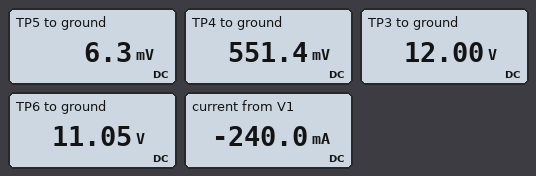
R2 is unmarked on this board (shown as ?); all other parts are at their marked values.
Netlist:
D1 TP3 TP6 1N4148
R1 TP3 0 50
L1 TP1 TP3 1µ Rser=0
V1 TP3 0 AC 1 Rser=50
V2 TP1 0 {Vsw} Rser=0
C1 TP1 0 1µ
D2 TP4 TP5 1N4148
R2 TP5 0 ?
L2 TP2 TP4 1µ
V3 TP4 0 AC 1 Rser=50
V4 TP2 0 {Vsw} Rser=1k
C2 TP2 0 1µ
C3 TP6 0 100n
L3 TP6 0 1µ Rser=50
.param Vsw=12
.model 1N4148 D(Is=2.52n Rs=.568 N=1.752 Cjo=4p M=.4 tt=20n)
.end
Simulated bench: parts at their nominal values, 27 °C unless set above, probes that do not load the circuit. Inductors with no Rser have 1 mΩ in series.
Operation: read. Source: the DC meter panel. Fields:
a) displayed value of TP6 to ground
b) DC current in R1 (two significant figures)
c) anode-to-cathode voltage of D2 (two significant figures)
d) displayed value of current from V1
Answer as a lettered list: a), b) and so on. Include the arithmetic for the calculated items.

a) 11.05 V
b) (12 V) / 50 Ω = 240 mA
c) 551.4 mV - 6.3 mV = 550 mV
d) -240.0 mA
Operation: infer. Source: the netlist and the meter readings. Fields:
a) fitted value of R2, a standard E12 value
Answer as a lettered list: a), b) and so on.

a) 15 Ω
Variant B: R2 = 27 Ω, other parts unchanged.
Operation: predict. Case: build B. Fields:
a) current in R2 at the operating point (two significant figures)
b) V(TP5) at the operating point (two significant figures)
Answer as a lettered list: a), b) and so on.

a) 390 µA
b) 11 mV
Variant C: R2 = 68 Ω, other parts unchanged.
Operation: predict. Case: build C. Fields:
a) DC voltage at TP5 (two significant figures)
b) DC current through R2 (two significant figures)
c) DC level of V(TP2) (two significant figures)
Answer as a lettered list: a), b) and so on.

a) 22 mV
b) 330 µA
c) 560 mV
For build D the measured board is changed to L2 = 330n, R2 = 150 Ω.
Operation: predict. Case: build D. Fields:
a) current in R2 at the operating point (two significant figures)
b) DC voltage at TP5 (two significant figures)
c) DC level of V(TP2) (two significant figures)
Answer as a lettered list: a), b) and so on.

a) 250 µA
b) 38 mV
c) 560 mV
